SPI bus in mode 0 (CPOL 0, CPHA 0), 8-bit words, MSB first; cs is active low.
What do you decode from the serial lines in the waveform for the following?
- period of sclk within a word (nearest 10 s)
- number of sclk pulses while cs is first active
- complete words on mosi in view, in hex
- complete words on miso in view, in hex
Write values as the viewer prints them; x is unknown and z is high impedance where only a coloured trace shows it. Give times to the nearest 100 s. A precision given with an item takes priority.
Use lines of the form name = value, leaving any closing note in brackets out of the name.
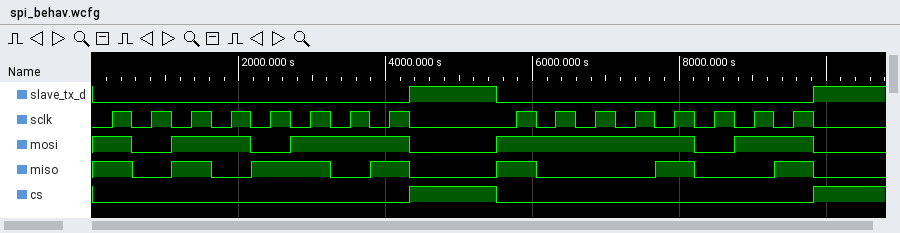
period of sclk within a word = 540 s
number of sclk pulses while cs is first active = 8
complete words on mosi in view, in hex = B7, FB
complete words on miso in view, in hex = AD, 89
